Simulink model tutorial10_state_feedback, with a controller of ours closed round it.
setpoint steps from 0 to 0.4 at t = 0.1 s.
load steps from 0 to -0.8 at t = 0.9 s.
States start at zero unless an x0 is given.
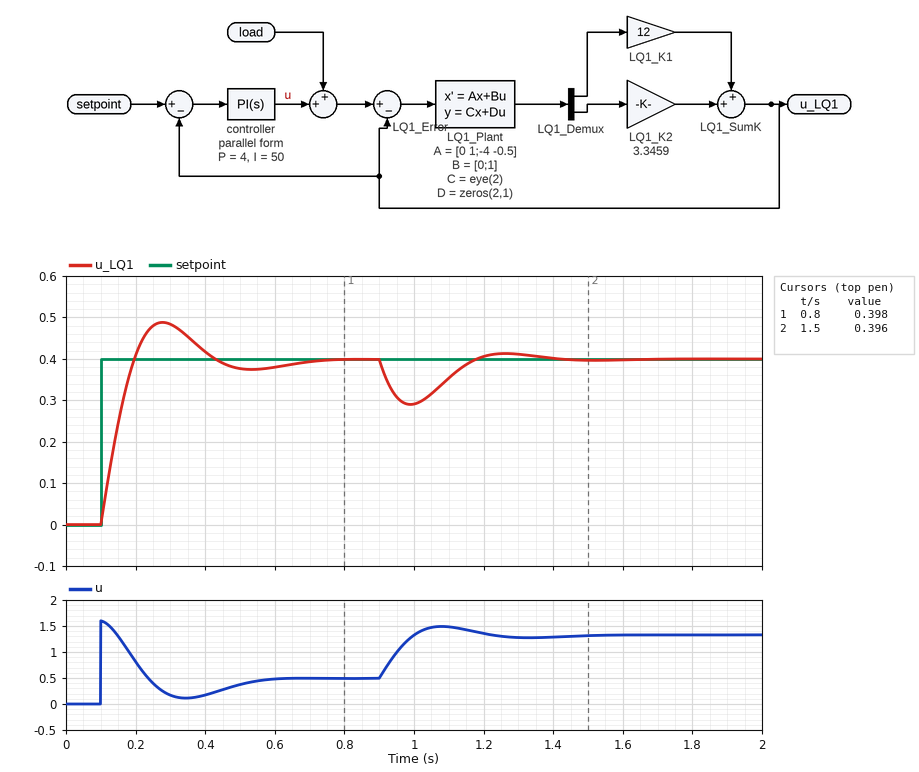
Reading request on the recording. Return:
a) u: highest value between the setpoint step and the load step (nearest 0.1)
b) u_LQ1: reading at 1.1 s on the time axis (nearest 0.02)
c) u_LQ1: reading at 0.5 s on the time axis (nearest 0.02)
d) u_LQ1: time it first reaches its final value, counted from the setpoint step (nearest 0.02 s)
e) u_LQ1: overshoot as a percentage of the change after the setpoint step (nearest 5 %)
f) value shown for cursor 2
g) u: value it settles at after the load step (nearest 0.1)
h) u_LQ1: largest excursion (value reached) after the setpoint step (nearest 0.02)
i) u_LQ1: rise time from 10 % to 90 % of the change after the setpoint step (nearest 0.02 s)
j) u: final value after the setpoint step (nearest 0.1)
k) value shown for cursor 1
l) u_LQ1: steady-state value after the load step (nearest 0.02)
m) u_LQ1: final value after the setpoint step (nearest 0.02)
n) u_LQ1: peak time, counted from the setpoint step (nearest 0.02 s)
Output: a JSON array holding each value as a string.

["1.6", "0.36", "0.38", "0.10 s", "20 %", "0.396", "1.3", "0.48", "0.08 s", "0.5", "0.398", "0.40", "0.40", "0.18 s"]
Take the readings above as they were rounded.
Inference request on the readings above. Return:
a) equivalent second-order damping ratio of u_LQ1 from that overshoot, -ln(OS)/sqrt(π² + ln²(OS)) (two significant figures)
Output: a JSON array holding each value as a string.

["0.46"]
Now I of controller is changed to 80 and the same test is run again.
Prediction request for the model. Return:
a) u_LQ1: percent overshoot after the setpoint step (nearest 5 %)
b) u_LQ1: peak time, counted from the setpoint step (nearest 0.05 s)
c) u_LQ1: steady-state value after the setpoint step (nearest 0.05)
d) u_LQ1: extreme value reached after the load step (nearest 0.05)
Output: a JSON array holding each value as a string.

["30 %", "0.15 s", "0.40", "0.30"]
